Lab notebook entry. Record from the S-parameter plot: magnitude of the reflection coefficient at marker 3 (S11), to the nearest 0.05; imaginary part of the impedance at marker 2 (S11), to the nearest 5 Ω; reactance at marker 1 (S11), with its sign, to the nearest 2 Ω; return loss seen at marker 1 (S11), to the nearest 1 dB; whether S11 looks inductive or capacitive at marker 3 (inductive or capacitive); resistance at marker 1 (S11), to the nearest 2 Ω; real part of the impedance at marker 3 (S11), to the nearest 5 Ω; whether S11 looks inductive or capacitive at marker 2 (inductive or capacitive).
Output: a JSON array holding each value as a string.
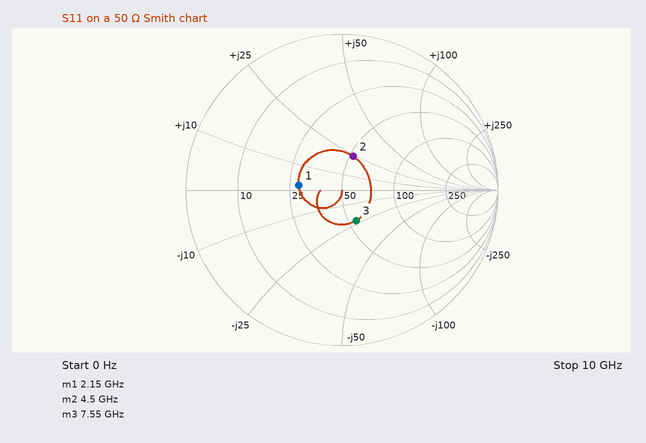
["0.20", "+25 Ω", "+2 Ω", "11 dB", "capacitive", "28 Ω", "55 Ω", "inductive"]
